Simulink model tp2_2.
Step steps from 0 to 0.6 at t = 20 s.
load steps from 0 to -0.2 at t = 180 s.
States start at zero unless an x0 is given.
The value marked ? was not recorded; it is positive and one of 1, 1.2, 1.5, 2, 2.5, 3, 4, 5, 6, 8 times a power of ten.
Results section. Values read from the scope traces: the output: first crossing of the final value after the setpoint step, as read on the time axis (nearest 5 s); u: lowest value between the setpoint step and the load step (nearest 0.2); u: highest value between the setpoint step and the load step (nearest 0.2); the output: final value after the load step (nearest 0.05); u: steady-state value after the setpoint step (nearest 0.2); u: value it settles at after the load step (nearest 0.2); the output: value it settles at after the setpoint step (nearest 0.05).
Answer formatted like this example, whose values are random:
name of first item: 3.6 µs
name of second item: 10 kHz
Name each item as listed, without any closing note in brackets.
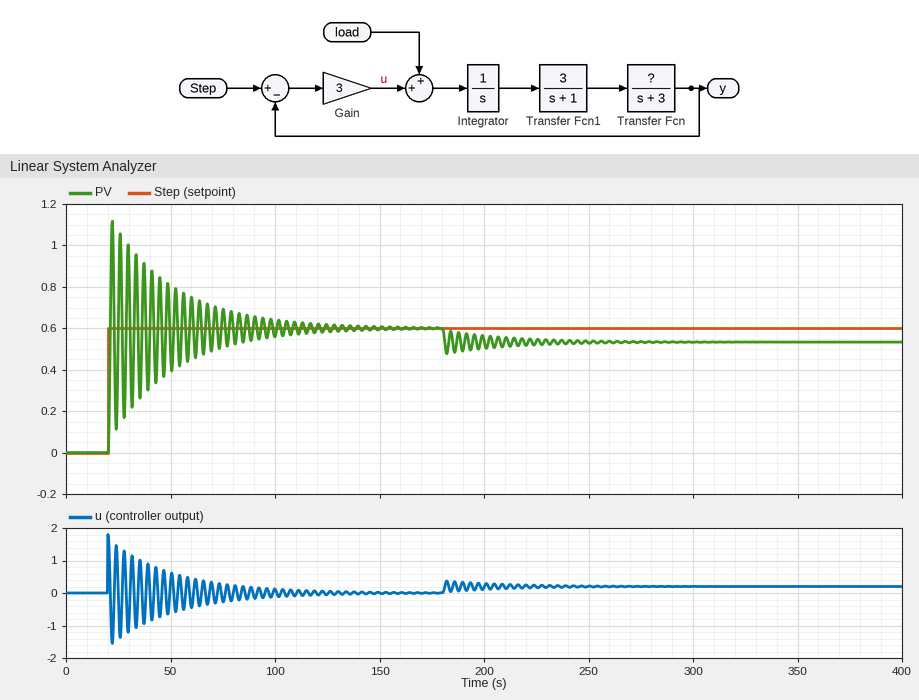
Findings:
the output: first crossing of the final value after the setpoint step, as read on the time axis: 20 s
u: lowest value between the setpoint step and the load step: -1.6
u: highest value between the setpoint step and the load step: 1.8
the output: final value after the load step: 0.55
u: steady-state value after the setpoint step: 0.0
u: value it settles at after the load step: 0.2
the output: value it settles at after the setpoint step: 0.60
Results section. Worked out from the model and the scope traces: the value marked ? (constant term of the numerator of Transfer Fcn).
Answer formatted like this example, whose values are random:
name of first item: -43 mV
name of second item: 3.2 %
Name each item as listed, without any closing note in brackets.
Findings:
the value marked ?: 1.2
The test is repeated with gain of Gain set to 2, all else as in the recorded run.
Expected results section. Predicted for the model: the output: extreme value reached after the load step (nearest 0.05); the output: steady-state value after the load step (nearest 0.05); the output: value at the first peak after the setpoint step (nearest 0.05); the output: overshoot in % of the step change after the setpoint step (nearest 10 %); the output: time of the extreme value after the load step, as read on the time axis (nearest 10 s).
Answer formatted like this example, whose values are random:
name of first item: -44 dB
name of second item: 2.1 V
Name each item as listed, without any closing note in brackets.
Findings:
the output: extreme value reached after the load step: 0.45
the output: steady-state value after the load step: 0.50
the output: value at the first peak after the setpoint step: 1.00
the output: overshoot in % of the step change after the setpoint step: 70 %
the output: time of the extreme value after the load step, as read on the time axis: 180 s
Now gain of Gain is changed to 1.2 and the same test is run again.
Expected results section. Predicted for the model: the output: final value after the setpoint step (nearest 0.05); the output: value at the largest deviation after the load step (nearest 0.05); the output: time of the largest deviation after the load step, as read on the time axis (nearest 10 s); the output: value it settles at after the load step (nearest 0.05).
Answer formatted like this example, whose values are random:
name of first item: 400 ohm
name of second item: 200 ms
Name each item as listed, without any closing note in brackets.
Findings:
the output: final value after the setpoint step: 0.60
the output: value at the largest deviation after the load step: 0.35
the output: time of the largest deviation after the load step, as read on the time axis: 180 s
the output: value it settles at after the load step: 0.45
